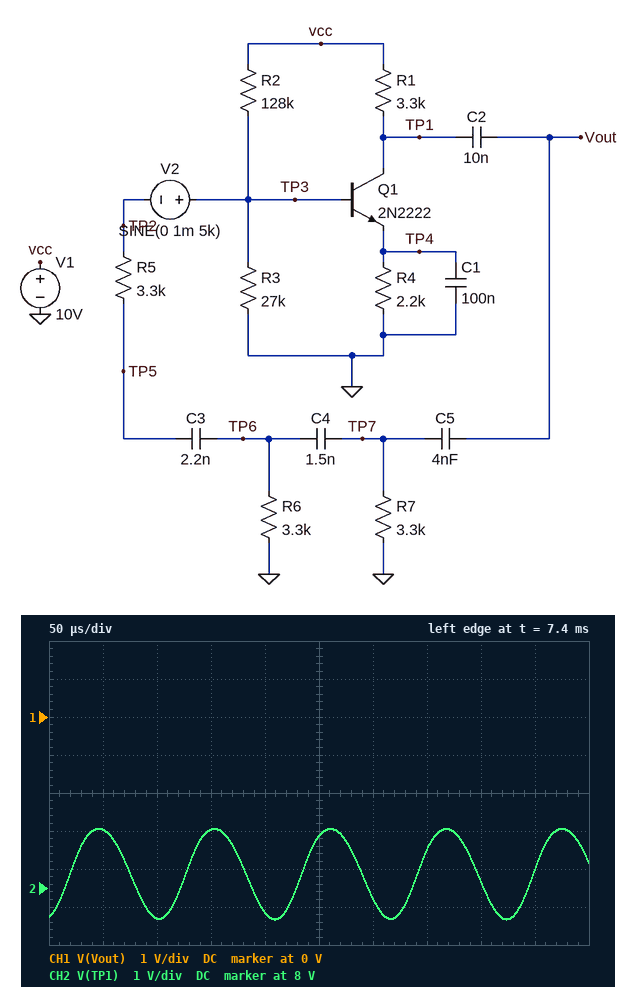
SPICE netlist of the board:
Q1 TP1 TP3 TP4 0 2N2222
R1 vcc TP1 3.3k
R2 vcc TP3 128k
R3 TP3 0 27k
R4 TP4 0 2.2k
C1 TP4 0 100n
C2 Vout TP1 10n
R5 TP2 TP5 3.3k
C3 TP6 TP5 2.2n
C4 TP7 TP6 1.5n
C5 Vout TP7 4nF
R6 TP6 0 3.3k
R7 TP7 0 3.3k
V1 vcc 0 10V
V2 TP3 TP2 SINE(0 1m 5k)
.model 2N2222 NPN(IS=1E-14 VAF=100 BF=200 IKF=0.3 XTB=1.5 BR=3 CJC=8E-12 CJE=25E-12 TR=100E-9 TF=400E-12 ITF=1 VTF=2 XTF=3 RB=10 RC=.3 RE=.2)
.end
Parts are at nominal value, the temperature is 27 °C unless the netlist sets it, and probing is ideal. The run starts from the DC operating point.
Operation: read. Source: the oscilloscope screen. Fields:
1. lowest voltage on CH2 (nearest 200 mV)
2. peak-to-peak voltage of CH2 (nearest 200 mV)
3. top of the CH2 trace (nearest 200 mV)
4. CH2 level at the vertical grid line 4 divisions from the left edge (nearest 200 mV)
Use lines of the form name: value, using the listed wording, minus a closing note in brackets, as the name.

lowest voltage on CH2: 7.2 V
peak-to-peak voltage of CH2: 2.4 V
top of the CH2 trace: 9.6 V
CH2 level at the vertical grid line 4 divisions from the left edge: 7.4 V
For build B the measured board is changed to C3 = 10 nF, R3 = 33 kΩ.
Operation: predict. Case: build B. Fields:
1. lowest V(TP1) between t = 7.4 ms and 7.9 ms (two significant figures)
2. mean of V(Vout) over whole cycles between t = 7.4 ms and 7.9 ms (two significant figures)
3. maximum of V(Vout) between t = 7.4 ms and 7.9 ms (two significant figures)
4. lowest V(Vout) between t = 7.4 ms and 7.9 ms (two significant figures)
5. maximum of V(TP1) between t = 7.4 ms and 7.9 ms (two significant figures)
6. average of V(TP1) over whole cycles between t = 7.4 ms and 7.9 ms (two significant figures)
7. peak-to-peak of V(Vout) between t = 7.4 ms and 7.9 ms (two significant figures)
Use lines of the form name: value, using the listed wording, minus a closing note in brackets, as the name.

lowest V(TP1) between t = 7.4 ms and 7.9 ms: 6.9 V
mean of V(Vout) over whole cycles between t = 7.4 ms and 7.9 ms: 5.7 V
maximum of V(Vout) between t = 7.4 ms and 7.9 ms: 6.6 V
lowest V(Vout) between t = 7.4 ms and 7.9 ms: 4.8 V
maximum of V(TP1) between t = 7.4 ms and 7.9 ms: 9.1 V
average of V(TP1) over whole cycles between t = 7.4 ms and 7.9 ms: 8.0 V
peak-to-peak of V(Vout) between t = 7.4 ms and 7.9 ms: 1.8 V
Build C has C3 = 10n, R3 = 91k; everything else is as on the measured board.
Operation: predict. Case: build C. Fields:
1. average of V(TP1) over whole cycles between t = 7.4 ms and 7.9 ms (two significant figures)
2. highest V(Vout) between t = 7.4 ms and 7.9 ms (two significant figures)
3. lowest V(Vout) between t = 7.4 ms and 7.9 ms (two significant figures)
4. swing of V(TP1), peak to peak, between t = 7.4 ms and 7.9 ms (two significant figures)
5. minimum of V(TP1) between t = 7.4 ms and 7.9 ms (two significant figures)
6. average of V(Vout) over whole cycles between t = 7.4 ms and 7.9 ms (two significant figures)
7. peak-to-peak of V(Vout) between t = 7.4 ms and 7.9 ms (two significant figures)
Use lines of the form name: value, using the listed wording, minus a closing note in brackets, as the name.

average of V(TP1) over whole cycles between t = 7.4 ms and 7.9 ms: 5.5 V
highest V(Vout) between t = 7.4 ms and 7.9 ms: 5.8 V
lowest V(Vout) between t = 7.4 ms and 7.9 ms: 2.0 V
swing of V(TP1), peak to peak, between t = 7.4 ms and 7.9 ms: 4.8 V
minimum of V(TP1) between t = 7.4 ms and 7.9 ms: 3.1 V
average of V(Vout) over whole cycles between t = 7.4 ms and 7.9 ms: 3.9 V
peak-to-peak of V(Vout) between t = 7.4 ms and 7.9 ms: 3.8 V
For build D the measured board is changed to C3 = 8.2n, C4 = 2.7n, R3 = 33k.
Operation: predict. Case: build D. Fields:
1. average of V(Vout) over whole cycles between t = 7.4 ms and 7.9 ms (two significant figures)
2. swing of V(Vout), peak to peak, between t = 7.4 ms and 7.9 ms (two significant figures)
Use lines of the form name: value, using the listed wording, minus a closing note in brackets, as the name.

average of V(Vout) over whole cycles between t = 7.4 ms and 7.9 ms: 5.7 V
swing of V(Vout), peak to peak, between t = 7.4 ms and 7.9 ms: 2.1 V
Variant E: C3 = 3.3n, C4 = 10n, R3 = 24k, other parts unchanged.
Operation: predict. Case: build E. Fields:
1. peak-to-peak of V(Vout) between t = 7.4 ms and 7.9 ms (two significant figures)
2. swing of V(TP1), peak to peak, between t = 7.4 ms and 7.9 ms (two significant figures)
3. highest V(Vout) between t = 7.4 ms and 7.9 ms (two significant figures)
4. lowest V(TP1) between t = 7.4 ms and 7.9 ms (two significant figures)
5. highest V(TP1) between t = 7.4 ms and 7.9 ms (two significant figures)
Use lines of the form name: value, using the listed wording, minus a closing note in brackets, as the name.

peak-to-peak of V(Vout) between t = 7.4 ms and 7.9 ms: 37 mV
swing of V(TP1), peak to peak, between t = 7.4 ms and 7.9 ms: 50 mV
highest V(Vout) between t = 7.4 ms and 7.9 ms: 6.2 V
lowest V(TP1) between t = 7.4 ms and 7.9 ms: 8.6 V
highest V(TP1) between t = 7.4 ms and 7.9 ms: 8.7 V
